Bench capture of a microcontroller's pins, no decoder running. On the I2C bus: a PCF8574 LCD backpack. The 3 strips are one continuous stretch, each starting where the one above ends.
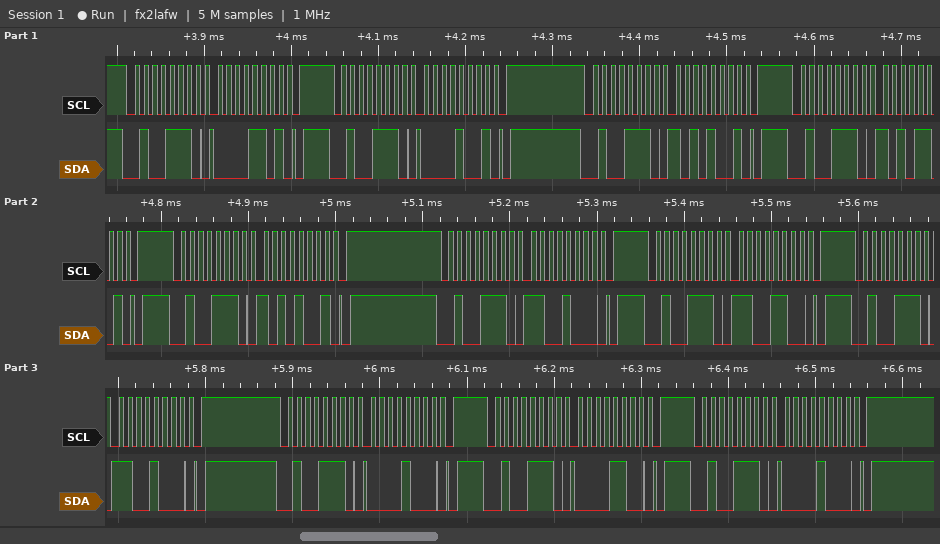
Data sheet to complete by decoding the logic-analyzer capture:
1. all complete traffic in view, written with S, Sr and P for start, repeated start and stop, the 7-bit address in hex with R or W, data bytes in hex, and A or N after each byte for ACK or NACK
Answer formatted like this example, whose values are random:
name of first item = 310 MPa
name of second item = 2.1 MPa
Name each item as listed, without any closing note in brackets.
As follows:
all complete traffic in view, written with S, Sr and P for start, repeated start and stop, the 7-bit address in hex with R or W, data bytes in hex, and A or N after each byte for ACK or NACK = S 27W A 0D A P S 27W A 09 A P S 27W A A9 A P S 27W A AD A P S 27W A A9 A P S 27W A C8 A P S 27W A CC A P S 27W A C8 A P S 27W A 08 A P S 27W A 0C A P S 27W A 08 A P
